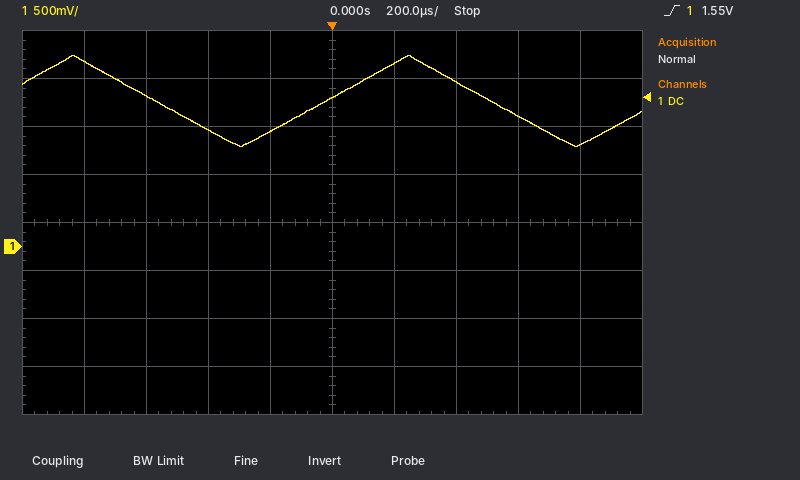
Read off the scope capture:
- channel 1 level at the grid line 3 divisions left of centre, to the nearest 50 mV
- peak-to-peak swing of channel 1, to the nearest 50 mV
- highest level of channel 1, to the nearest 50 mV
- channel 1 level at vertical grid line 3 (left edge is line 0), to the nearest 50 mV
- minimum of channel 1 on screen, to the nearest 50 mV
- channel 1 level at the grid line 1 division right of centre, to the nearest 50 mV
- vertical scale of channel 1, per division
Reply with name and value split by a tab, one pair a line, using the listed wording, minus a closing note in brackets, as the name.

channel 1 level at the grid line 3 divisions left of centre, to the nearest 50 mV	1.55 V
peak-to-peak swing of channel 1, to the nearest 50 mV	950 mV
highest level of channel 1, to the nearest 50 mV	2.00 V
channel 1 level at vertical grid line 3 (left edge is line 0), to the nearest 50 mV	1.20 V
minimum of channel 1 on screen, to the nearest 50 mV	1.05 V
channel 1 level at the grid line 1 division right of centre, to the nearest 50 mV	1.90 V
vertical scale of channel 1, per division	500 mV
